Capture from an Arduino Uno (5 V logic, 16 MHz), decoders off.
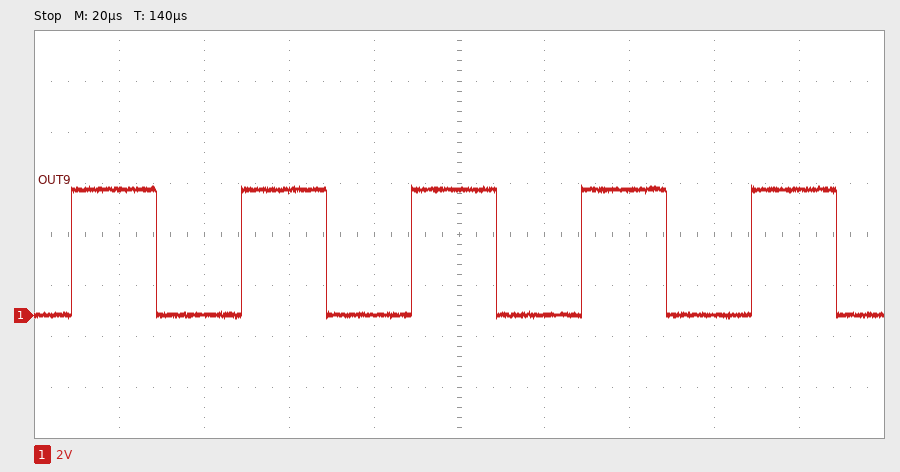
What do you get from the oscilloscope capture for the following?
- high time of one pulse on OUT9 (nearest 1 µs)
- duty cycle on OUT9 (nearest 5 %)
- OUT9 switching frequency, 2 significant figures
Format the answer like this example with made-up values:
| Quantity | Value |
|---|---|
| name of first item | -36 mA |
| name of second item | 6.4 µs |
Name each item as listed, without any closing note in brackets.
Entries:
| Quantity | Value |
|---|---|
| high time of one pulse on OUT9 | 20 µs |
| duty cycle on OUT9 | 50 % |
| OUT9 switching frequency, 2 significant figures | 25 kHz |
